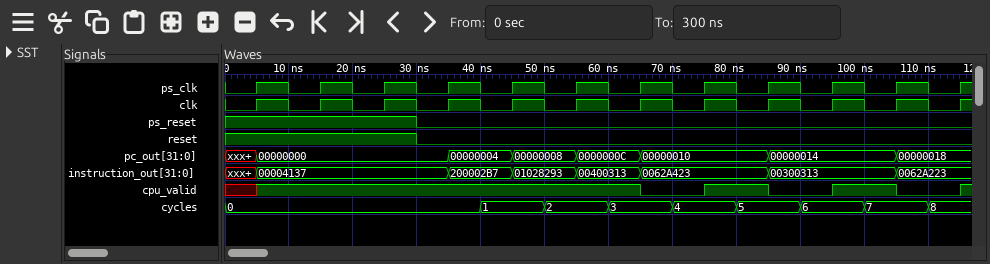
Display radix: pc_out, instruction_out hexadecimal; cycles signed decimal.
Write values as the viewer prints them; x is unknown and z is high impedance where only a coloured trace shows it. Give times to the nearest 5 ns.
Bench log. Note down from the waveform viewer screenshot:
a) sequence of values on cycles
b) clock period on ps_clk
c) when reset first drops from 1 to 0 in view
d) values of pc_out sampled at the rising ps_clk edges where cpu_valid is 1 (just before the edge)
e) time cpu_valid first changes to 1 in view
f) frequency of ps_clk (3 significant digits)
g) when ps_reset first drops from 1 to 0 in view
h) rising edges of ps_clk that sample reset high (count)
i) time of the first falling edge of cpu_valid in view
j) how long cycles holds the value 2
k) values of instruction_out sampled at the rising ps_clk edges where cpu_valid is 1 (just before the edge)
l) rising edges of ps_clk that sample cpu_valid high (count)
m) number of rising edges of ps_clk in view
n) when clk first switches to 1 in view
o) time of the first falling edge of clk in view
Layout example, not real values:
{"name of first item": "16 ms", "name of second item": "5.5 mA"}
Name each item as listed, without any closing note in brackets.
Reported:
{"sequence of values on cycles": "0, 1, 2, 3, 4, 5, 6, 7, 8", "clock period on ps_clk": "10 ns", "when reset first drops from 1 to 0 in view": "30 ns", "values of pc_out sampled at the rising ps_clk edges where cpu_valid is 1": "00000000, 00000000, 00000000, 00000004, 00000008, 0000000C, 00000010, 00000014", "time cpu_valid first changes to 1 in view": "5 ns", "frequency of ps_clk": "100 MHz", "when ps_reset first drops from 1 to 0 in view": "30 ns", "rising edges of ps_clk that sample reset high": "3", "time of the first falling edge of cpu_valid in view": "65 ns", "how long cycles holds the value 2": "10 ns", "values of instruction_out sampled at the rising ps_clk edges where cpu_valid is 1": "00004137, 00004137, 00004137, 200002B7, 01028293, 00400313, 0062A423, 00300313", "rising edges of ps_clk that sample cpu_valid high": "8", "number of rising edges of ps_clk in view": "12", "when clk first switches to 1 in view": "5 ns", "time of the first falling edge of clk in view": "10 ns"}
